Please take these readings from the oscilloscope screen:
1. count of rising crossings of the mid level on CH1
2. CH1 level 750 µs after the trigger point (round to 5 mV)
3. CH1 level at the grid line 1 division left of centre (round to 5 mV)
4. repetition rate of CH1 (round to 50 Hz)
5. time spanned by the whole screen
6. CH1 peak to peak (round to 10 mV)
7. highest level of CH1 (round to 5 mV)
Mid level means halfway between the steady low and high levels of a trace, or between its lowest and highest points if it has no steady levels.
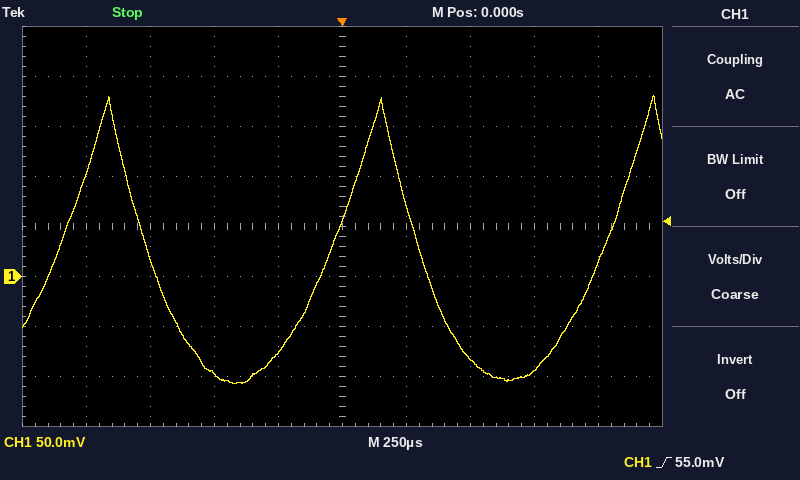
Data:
3
-95 mV
-75 mV
950 Hz
2.5 ms
290 mV
180 mV
